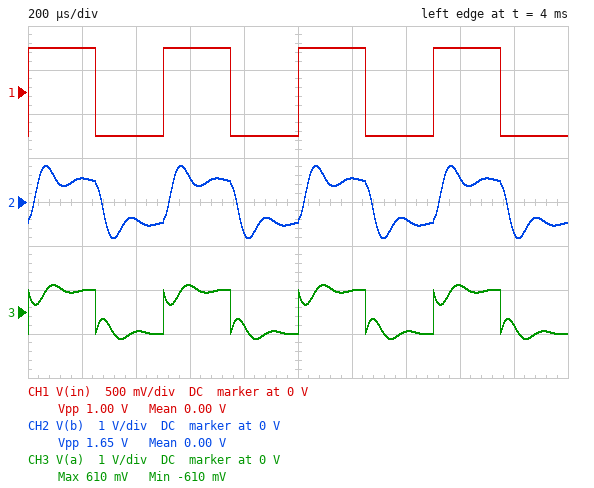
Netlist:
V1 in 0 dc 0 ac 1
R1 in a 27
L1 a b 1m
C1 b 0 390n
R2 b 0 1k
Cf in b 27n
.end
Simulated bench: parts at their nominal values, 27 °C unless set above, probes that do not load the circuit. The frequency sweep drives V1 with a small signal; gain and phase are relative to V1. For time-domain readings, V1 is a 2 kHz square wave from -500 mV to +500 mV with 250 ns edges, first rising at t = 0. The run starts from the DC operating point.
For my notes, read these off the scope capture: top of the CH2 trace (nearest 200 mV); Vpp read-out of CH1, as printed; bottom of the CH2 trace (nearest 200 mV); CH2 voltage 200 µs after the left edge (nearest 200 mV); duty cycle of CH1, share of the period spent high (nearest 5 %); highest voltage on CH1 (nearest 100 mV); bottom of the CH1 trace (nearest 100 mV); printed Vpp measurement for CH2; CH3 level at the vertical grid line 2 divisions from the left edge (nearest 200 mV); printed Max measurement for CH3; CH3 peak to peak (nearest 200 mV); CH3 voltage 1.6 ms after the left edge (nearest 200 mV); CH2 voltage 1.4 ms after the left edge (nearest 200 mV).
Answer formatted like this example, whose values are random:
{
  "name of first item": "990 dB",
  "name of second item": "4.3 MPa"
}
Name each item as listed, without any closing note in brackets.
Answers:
{
  "top of the CH2 trace": "800 mV",
  "Vpp read-out of CH1, as printed": "1.00 V",
  "bottom of the CH2 trace": "-800 mV",
  "CH2 voltage 200 µs after the left edge": "600 mV",
  "duty cycle of CH1, share of the period spent high": "50 %",
  "highest voltage on CH1": "500 mV",
  "bottom of the CH1 trace": "-500 mV",
  "printed Vpp measurement for CH2": "1.65 V",
  "CH3 level at the vertical grid line 2 divisions from the left edge": "-400 mV",
  "printed Max measurement for CH3": "610 mV",
  "CH3 peak to peak": "1.2 V",
  "CH3 voltage 1.6 ms after the left edge": "600 mV",
  "CH2 voltage 1.4 ms after the left edge": "-400 mV"
}
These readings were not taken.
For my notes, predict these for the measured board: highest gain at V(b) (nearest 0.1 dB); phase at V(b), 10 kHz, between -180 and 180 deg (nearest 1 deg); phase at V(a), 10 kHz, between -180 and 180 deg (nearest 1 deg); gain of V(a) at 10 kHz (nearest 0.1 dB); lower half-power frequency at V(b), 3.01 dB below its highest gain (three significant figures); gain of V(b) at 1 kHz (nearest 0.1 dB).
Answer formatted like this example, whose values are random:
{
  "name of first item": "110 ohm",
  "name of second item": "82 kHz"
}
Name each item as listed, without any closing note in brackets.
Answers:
{
  "highest gain at V(b)": "4.2 dB",
  "phase at V(b), 10 kHz, between -180 and 180 deg": "-126 deg",
  "phase at V(a), 10 kHz, between -180 and 180 deg": "42 deg",
  "gain of V(a) at 10 kHz": "-3.6 dB",
  "lower half-power frequency at V(b), 3.01 dB below its highest gain": "3.64 kHz",
  "gain of V(b) at 1 kHz": "-0.1 dB"
}
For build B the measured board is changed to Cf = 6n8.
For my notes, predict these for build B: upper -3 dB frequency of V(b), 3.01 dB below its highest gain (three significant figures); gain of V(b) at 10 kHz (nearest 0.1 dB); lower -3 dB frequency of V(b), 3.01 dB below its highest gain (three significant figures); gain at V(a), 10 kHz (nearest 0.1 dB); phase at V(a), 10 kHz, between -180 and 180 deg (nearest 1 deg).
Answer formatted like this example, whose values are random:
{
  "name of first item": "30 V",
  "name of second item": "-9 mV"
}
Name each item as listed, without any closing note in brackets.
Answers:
{
  "upper -3 dB frequency of V(b), 3.01 dB below its highest gain": "9.50 kHz",
  "gain of V(b) at 10 kHz": "0.6 dB",
  "lower -3 dB frequency of V(b), 3.01 dB below its highest gain": "4.17 kHz",
  "gain at V(a), 10 kHz": "-4.1 dB",
  "phase at V(a), 10 kHz, between -180 and 180 deg": "46 deg"
}
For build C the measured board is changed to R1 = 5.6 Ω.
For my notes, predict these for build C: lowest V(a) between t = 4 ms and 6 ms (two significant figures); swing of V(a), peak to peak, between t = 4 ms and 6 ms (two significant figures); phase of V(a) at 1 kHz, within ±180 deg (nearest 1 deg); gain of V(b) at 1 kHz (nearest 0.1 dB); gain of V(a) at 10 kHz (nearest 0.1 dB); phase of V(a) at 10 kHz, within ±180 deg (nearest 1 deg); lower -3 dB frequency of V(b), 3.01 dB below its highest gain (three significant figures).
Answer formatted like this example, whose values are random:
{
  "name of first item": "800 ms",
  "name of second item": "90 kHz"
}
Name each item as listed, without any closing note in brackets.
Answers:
{
  "lowest V(a) between t = 4 ms and 6 ms": "-550 mV",
  "swing of V(a), peak to peak, between t = 4 ms and 6 ms": "1.1 V",
  "phase of V(a) at 1 kHz, within ±180 deg": "-1 deg",
  "gain of V(b) at 1 kHz": "0.1 dB",
  "gain of V(a) at 10 kHz": "-0.3 dB",
  "phase of V(a) at 10 kHz, within ±180 deg": "12 deg",
  "lower -3 dB frequency of V(b), 3.01 dB below its highest gain": "7.08 kHz"
}
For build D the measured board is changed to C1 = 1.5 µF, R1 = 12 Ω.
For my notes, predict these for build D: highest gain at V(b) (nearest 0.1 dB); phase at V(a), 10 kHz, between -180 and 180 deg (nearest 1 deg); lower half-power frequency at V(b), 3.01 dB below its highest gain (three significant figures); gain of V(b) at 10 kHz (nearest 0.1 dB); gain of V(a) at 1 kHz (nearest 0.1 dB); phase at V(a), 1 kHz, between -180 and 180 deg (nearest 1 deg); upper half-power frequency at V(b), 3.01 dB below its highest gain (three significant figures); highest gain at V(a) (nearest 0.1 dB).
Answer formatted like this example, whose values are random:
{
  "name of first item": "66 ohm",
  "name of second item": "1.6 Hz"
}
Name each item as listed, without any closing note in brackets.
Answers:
{
  "highest gain at V(b)": "6.2 dB",
  "phase at V(a), 10 kHz, between -180 and 180 deg": "13 deg",
  "lower half-power frequency at V(b), 3.01 dB below its highest gain": "2.57 kHz",
  "gain of V(b) at 10 kHz": "-15.2 dB",
  "gain of V(a) at 1 kHz": "-0.2 dB",
  "phase at V(a), 1 kHz, between -180 and 180 deg": "-7 deg",
  "upper half-power frequency at V(b), 3.01 dB below its highest gain": "4.76 kHz",
  "highest gain at V(a)": "0 dB"
}
